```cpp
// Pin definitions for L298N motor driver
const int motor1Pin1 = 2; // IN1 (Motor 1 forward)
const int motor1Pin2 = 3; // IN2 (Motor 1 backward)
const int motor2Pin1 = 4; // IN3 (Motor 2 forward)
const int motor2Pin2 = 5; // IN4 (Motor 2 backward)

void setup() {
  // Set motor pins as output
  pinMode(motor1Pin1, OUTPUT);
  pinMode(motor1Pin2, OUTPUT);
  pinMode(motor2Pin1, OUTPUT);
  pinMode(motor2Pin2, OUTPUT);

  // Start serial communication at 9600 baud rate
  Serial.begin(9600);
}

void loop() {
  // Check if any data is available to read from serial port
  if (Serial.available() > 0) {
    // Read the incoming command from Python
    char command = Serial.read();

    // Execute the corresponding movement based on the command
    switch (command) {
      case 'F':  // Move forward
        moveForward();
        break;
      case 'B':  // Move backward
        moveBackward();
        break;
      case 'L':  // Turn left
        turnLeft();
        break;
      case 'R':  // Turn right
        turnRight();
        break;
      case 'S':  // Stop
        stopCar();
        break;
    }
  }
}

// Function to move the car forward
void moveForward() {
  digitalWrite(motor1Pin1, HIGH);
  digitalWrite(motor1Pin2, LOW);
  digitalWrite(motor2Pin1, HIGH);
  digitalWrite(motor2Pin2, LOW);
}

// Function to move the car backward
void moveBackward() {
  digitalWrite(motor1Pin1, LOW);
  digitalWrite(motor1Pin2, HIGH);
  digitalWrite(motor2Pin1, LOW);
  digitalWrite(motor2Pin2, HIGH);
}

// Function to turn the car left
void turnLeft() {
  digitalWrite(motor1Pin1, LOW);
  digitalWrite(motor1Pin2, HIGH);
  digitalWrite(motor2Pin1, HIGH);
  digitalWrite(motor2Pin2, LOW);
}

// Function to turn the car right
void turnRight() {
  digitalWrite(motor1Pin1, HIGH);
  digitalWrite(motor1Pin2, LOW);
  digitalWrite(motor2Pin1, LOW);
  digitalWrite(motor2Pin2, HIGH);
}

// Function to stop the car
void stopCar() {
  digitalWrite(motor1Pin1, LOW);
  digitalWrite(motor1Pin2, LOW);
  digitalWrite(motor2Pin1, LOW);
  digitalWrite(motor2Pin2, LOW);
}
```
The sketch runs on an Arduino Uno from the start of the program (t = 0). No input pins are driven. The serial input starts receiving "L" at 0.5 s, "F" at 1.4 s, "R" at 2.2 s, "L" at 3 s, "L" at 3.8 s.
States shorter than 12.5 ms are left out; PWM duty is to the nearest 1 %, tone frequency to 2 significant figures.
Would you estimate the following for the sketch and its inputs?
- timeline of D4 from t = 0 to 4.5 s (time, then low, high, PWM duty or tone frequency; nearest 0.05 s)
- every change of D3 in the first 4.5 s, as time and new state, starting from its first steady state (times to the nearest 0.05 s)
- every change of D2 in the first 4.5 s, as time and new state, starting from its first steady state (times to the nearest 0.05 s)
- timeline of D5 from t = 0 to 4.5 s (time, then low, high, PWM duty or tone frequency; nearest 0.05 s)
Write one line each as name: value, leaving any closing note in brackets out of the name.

timeline of D4 from t = 0 to 4.5 s: 0 s low; 0.5 s high; 2.2 s low; 3 s high
every change of D3 in the first 4.5 s, as time and new state, starting from its first steady state: 0 s low; 0.5 s high; 1.4 s low; 3 s high
every change of D2 in the first 4.5 s, as time and new state, starting from its first steady state: 0 s low; 1.4 s high; 3 s low
timeline of D5 from t = 0 to 4.5 s: 0 s low; 2.2 s high; 3 s low
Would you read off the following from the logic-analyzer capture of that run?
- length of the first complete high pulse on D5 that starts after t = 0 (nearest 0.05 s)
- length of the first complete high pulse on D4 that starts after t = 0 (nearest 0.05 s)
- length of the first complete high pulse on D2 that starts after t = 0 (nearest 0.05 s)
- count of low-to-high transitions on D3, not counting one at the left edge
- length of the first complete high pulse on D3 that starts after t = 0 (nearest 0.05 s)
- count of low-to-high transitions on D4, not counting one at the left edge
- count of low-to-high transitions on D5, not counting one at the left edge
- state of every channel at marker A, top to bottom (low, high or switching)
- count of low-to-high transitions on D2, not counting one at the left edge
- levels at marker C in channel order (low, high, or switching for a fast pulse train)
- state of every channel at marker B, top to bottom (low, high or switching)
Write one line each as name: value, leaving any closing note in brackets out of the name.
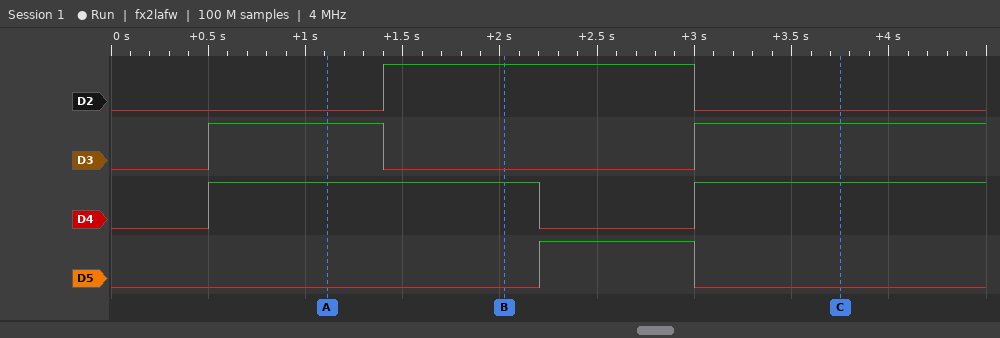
length of the first complete high pulse on D5 that starts after t = 0: 0.80 s
length of the first complete high pulse on D4 that starts after t = 0: 1.70 s
length of the first complete high pulse on D2 that starts after t = 0: 1.60 s
count of low-to-high transitions on D3, not counting one at the left edge: 2
length of the first complete high pulse on D3 that starts after t = 0: 0.90 s
count of low-to-high transitions on D4, not counting one at the left edge: 2
count of low-to-high transitions on D5, not counting one at the left edge: 1
state of every channel at marker A, top to bottom: D2 low, D3 high, D4 high, D5 low
count of low-to-high transitions on D2, not counting one at the left edge: 1
levels at marker C in channel order: D2 low, D3 high, D4 high, D5 low
state of every channel at marker B, top to bottom: D2 high, D3 low, D4 high, D5 low
